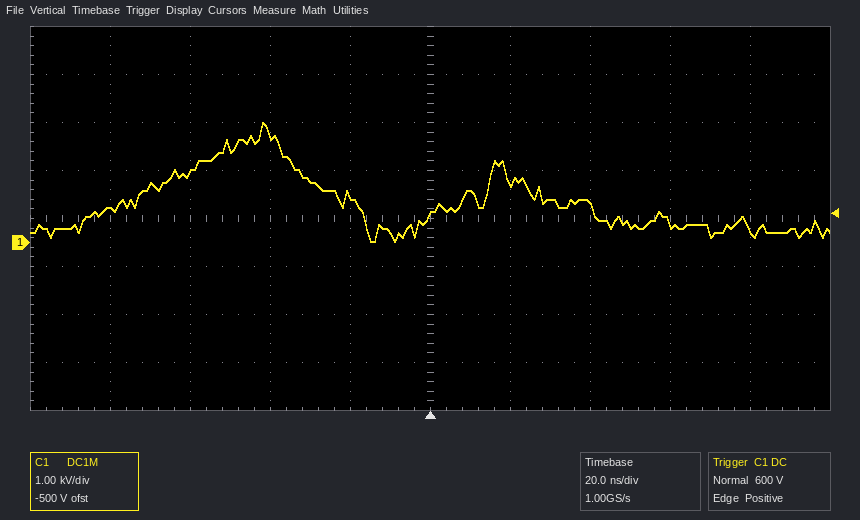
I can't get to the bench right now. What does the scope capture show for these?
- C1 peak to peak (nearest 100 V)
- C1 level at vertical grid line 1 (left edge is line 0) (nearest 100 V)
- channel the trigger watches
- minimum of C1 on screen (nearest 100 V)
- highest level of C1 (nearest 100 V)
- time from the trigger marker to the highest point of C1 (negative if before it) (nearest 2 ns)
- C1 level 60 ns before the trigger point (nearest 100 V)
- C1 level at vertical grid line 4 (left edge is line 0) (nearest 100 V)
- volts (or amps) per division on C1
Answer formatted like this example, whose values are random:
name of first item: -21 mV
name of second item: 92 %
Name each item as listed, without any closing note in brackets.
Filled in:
C1 peak to peak: 2.5 kV
C1 level at vertical grid line 1 (left edge is line 0): 700 V
channel the trigger watches: C1
minimum of C1 on screen: 0.0 kV
highest level of C1: 2.5 kV
time from the trigger marker to the highest point of C1 (negative if before it): -42 ns
C1 level 60 ns before the trigger point: 1.4 kV
C1 level at vertical grid line 4 (left edge is line 0): 1.0 kV
volts (or amps) per division on C1: 1 kV
